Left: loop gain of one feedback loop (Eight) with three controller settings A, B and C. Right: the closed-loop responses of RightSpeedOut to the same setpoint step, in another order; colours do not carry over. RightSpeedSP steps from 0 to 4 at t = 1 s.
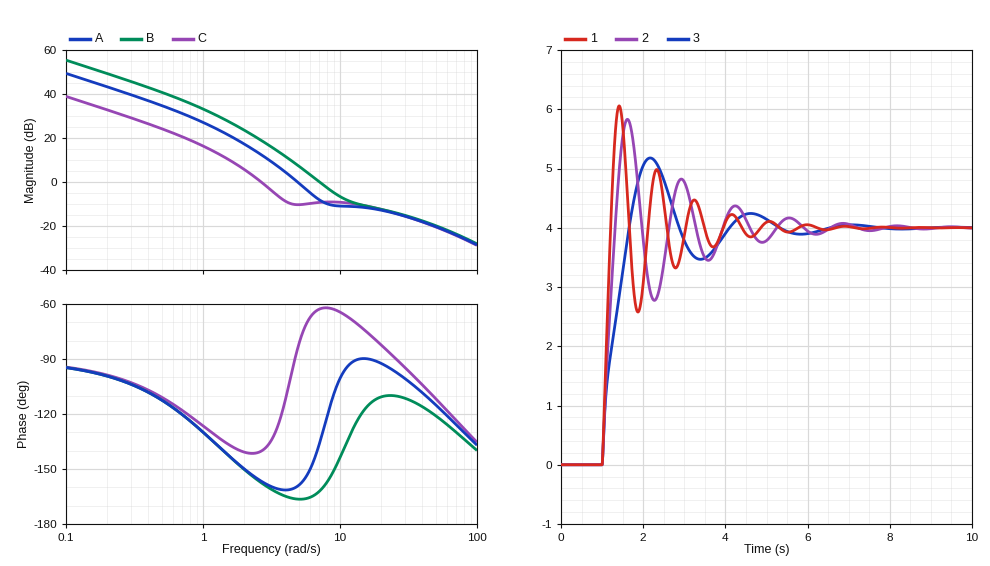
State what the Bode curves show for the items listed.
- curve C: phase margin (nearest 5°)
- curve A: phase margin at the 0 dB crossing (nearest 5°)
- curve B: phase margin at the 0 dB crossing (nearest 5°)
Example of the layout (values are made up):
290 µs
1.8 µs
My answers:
40°
20°
20°
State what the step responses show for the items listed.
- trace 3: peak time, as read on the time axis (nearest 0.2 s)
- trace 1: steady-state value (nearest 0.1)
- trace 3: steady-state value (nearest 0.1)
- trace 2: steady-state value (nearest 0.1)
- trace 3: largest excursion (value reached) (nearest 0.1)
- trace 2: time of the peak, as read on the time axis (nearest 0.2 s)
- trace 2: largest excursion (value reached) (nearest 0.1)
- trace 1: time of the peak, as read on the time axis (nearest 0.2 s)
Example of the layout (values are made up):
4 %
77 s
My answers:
2.2 s
4.0
4.0
4.0
5.2
1.6 s
5.8
1.4 s
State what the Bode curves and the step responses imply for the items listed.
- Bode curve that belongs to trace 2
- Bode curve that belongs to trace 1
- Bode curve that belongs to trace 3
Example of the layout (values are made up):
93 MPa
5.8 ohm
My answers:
A
B
C
